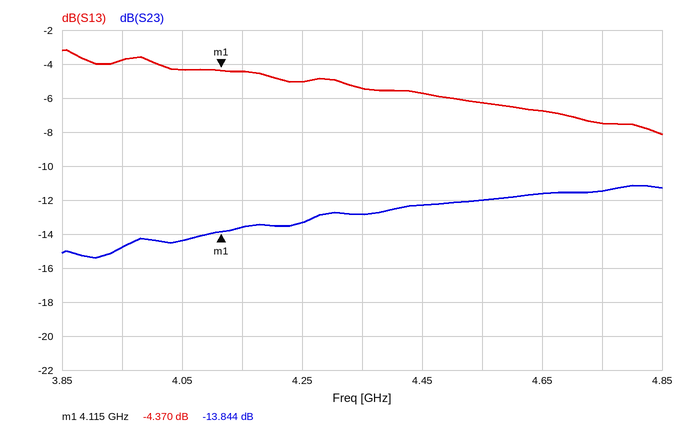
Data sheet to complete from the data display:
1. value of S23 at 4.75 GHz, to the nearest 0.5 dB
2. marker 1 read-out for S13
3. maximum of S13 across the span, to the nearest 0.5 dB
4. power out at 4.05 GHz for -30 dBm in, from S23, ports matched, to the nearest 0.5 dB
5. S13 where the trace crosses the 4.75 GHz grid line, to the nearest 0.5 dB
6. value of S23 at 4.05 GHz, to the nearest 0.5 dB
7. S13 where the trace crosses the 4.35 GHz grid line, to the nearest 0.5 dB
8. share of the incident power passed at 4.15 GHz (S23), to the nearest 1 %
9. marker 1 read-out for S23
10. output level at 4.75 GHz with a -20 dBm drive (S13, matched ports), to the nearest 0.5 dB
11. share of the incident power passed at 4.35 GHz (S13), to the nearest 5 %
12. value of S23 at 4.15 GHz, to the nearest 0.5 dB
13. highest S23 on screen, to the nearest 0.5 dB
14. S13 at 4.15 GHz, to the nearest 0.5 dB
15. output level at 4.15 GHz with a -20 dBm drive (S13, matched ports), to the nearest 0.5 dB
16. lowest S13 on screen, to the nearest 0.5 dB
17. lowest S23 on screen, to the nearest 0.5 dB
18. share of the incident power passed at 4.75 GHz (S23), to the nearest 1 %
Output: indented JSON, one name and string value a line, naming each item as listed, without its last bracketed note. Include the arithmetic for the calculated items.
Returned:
{
  "value of S23 at 4.75 GHz, to the nearest 0.5 dB": "-11.5 dB",
  "marker 1 read-out for S13": "-4.370 dB",
  "maximum of S13 across the span, to the nearest 0.5 dB": "-3.0 dB",
  "power out at 4.05 GHz for -30 dBm in, from S23, ports matched, to the nearest 0.5 dB": "-30 dBm + (-14.5 dB) = -44.5 dBm",
  "S13 where the trace crosses the 4.75 GHz grid line, to the nearest 0.5 dB": "-7.5 dB",
  "value of S23 at 4.05 GHz, to the nearest 0.5 dB": "-14.5 dB",
  "S13 where the trace crosses the 4.35 GHz grid line, to the nearest 0.5 dB": "-5.5 dB",
  "share of the incident power passed at 4.15 GHz (S23), to the nearest 1 %": "10^(-13.5/10) ≈ 4 %",
  "marker 1 read-out for S23": "-13.844 dB",
  "output level at 4.75 GHz with a -20 dBm drive (S13, matched ports), to the nearest 0.5 dB": "-20 dBm + (-7.5 dB) = -27.5 dBm",
  "share of the incident power passed at 4.35 GHz (S13), to the nearest 5 %": "10^(-5.5/10) ≈ 28.2 %, so 30 % to the nearest 5 %",
  "value of S23 at 4.15 GHz, to the nearest 0.5 dB": "-13.5 dB",
  "highest S23 on screen, to the nearest 0.5 dB": "-11.0 dB",
  "S13 at 4.15 GHz, to the nearest 0.5 dB": "-4.5 dB",
  "output level at 4.15 GHz with a -20 dBm drive (S13, matched ports), to the nearest 0.5 dB": "-20 dBm + (-4.5 dB) = -24.5 dBm",
  "lowest S13 on screen, to the nearest 0.5 dB": "-8.0 dB",
  "lowest S23 on screen, to the nearest 0.5 dB": "-15.5 dB",
  "share of the incident power passed at 4.75 GHz (S23), to the nearest 1 %": "10^(-11.5/10) ≈ 7 %"
}
